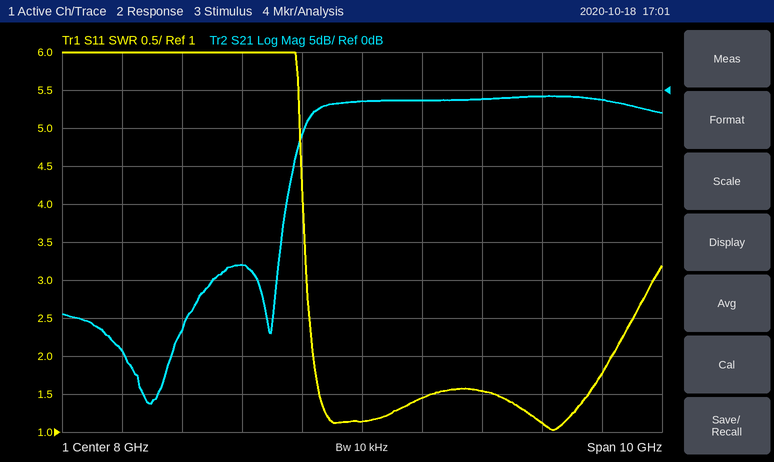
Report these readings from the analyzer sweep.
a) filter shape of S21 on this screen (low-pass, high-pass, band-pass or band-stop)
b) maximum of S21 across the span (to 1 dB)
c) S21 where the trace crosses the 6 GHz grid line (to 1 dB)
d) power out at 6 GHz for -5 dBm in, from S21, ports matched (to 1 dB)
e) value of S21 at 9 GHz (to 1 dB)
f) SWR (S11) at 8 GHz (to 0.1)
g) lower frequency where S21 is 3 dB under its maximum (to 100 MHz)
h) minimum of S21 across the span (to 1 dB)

high-pass
-1 dB
-23 dB
-28 dBm
-1 dB
1.1
7.1 GHz
-41 dB
